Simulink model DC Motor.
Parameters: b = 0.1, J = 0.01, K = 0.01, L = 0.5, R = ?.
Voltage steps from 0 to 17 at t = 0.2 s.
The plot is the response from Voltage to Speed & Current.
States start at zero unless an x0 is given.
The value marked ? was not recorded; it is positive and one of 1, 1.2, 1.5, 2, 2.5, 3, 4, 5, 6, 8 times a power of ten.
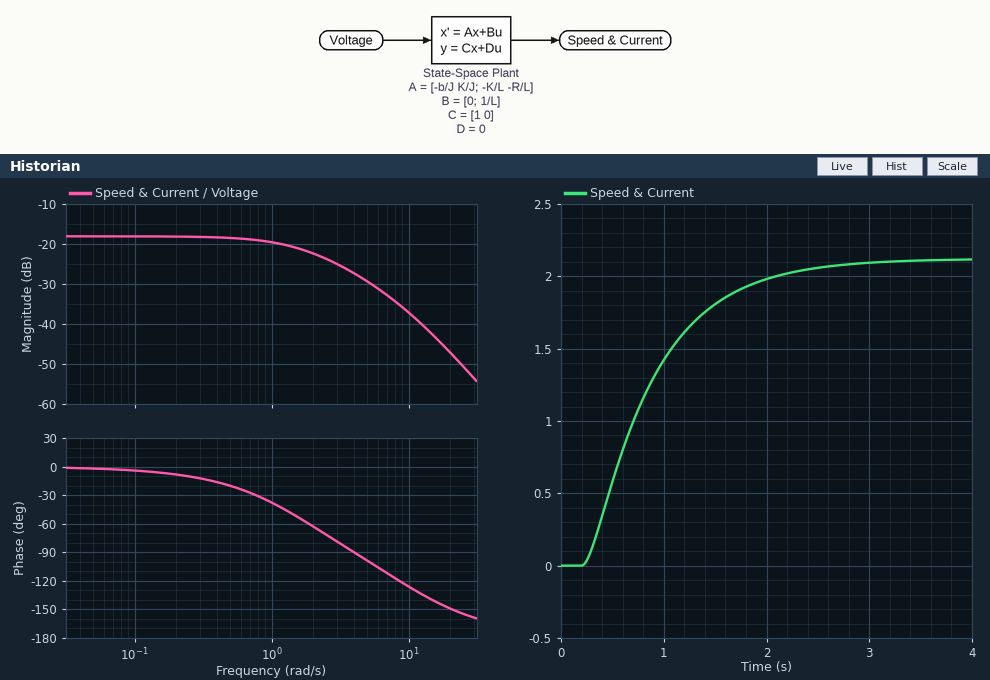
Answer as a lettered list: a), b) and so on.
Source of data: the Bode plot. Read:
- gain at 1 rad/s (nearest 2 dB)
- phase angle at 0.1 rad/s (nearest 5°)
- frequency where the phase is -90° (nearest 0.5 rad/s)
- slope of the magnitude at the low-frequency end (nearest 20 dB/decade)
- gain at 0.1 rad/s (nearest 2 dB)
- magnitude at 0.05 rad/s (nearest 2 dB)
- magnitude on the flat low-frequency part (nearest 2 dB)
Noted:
a) -20 dB
b) -5°
c) 4.0 rad/s
d) 0 dB/decade
e) -18 dB
f) -18 dB
g) -18 dB
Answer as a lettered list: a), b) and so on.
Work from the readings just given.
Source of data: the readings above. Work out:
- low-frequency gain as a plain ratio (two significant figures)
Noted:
a) 0.13
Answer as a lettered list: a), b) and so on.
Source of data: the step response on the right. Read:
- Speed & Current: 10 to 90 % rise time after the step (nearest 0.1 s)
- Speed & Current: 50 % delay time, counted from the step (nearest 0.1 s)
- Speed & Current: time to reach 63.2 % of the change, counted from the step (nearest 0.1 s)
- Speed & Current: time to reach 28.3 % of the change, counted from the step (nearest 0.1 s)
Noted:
a) 1.4 s
b) 0.5 s
c) 0.7 s
d) 0.3 s
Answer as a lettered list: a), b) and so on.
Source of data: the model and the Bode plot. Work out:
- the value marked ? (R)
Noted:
a) 0.8
